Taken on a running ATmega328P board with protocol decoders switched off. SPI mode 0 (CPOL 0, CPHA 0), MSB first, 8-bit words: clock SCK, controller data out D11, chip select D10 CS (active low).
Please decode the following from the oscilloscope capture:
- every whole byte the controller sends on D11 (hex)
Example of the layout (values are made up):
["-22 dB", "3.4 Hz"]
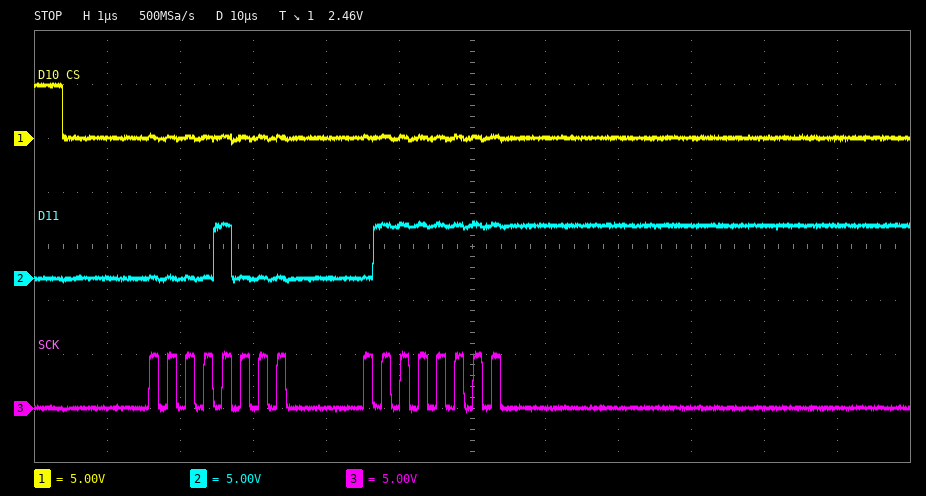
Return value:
["0x08 0x7F"]
